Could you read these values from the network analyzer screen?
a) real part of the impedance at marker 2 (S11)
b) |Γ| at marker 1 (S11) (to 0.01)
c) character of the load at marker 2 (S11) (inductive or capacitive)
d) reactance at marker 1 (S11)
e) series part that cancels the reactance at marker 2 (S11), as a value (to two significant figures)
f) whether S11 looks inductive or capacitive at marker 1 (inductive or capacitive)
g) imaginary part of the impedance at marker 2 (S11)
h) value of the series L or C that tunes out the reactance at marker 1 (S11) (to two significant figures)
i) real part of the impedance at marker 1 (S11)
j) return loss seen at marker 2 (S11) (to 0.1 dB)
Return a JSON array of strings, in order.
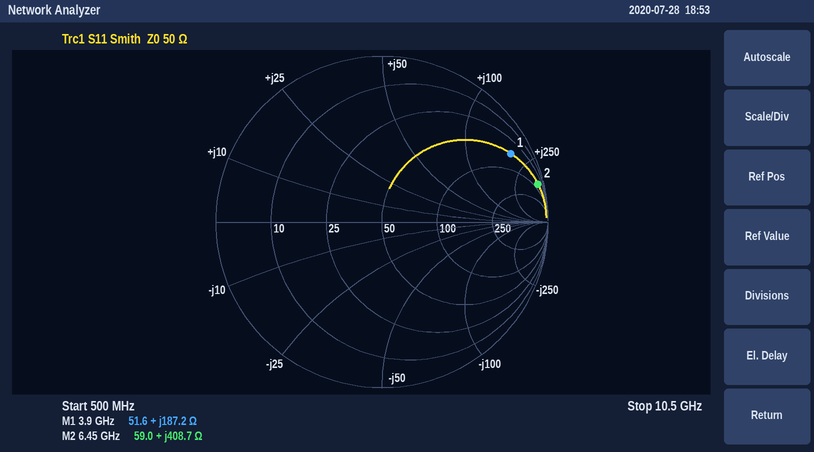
["59.0 Ω", "0.88", "inductive", "+187.2 Ω", "60 fF", "inductive", "+408.7 Ω", "220 fF", "51.6 Ω", "0.3 dB"]
